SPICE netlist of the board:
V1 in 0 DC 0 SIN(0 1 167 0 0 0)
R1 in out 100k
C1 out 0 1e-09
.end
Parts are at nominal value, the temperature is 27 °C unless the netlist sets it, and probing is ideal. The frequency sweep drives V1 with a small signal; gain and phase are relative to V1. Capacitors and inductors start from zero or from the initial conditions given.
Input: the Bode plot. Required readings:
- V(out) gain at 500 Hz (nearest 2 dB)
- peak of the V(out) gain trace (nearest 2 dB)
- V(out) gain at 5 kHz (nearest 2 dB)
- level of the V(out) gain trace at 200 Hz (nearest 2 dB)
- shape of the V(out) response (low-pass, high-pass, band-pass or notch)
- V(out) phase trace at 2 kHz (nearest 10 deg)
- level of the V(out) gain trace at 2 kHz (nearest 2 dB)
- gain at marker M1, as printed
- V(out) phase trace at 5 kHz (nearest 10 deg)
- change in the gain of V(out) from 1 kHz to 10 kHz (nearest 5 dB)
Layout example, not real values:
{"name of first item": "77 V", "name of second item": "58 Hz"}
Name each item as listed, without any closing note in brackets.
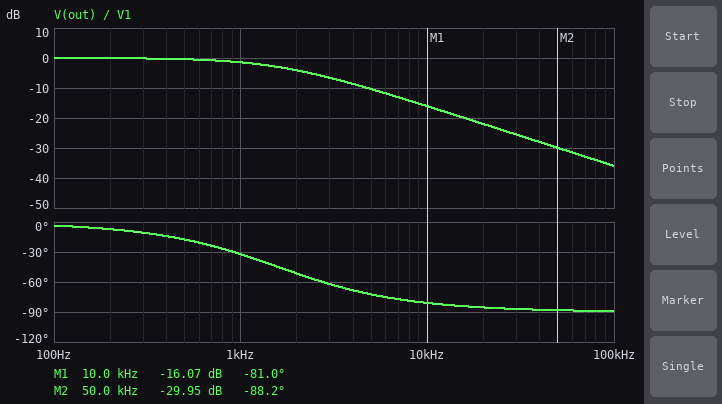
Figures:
{"V(out) gain at 500 Hz": "0 dB", "peak of the V(out) gain trace": "0 dB", "V(out) gain at 5 kHz": "-10 dB", "level of the V(out) gain trace at 200 Hz": "0 dB", "shape of the V(out) response": "low-pass", "V(out) phase trace at 2 kHz": "-50 deg", "level of the V(out) gain trace at 2 kHz": "-4 dB", "gain at marker M1, as printed": "-16.07 dB", "V(out) phase trace at 5 kHz": "-70 deg", "change in the gain of V(out) from 1 kHz to 10 kHz": "-15 dB"}
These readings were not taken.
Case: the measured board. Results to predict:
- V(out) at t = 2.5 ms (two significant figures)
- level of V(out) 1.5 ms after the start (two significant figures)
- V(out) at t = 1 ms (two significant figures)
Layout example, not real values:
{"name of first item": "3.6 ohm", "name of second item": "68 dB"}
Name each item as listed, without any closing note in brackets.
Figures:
{"V(out) at t = 2.5 ms": "580 mV", "level of V(out) 1.5 ms after the start": "990 mV", "V(out) at t = 1 ms": "810 mV"}
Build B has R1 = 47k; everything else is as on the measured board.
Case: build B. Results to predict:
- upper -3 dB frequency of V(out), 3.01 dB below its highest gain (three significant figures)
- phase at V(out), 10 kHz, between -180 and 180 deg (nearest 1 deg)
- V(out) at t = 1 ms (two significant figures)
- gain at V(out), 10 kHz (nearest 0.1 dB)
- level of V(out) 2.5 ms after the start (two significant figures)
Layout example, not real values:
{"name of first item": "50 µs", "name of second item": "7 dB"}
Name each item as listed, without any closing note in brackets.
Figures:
{"upper -3 dB frequency of V(out), 3.01 dB below its highest gain": "3.39 kHz", "phase at V(out), 10 kHz, between -180 and 180 deg": "-71 deg", "V(out) at t = 1 ms": "840 mV", "gain at V(out), 10 kHz": "-9.9 dB", "level of V(out) 2.5 ms after the start": "540 mV"}
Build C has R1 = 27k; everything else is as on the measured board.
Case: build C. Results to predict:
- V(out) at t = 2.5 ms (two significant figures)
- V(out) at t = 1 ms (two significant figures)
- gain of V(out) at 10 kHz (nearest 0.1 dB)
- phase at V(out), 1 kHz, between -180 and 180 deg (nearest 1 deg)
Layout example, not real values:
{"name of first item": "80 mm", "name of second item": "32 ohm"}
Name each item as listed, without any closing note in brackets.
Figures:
{"V(out) at t = 2.5 ms": "520 mV", "V(out) at t = 1 ms": "850 mV", "gain of V(out) at 10 kHz": "-5.9 dB", "phase at V(out), 1 kHz, between -180 and 180 deg": "-10 deg"}
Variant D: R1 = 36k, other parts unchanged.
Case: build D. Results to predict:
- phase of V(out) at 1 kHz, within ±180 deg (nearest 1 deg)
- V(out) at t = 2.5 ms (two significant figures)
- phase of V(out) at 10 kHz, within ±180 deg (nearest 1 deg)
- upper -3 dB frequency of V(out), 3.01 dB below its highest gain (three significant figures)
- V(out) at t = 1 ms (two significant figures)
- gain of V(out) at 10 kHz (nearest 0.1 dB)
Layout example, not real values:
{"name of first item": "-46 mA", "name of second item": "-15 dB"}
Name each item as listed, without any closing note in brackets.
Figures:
{"phase of V(out) at 1 kHz, within ±180 deg": "-13 deg", "V(out) at t = 2.5 ms": "530 mV", "phase of V(out) at 10 kHz, within ±180 deg": "-66 deg", "upper -3 dB frequency of V(out), 3.01 dB below its highest gain": "4.42 kHz", "V(out) at t = 1 ms": "850 mV", "gain of V(out) at 10 kHz": "-7.9 dB"}
